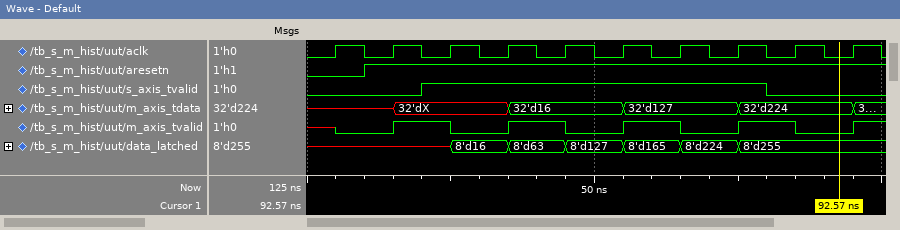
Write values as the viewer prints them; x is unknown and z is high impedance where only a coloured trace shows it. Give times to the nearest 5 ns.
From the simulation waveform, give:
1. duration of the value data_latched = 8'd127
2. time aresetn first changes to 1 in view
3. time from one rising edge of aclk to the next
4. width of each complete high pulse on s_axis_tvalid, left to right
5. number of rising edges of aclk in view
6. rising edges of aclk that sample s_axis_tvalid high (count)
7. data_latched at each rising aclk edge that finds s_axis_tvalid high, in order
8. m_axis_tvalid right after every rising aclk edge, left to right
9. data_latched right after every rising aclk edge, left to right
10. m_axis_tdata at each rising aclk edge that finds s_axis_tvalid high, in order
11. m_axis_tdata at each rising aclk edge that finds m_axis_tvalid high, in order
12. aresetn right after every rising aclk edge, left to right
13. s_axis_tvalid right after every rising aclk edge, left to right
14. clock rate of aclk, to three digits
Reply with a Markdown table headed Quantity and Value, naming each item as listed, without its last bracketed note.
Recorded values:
| Quantity | Value |
|---|---|
| duration of the value data_latched = 8'd127 | 10 ns |
| time aresetn first changes to 1 in view | 10 ns |
| time from one rising edge of aclk to the next | 10 ns |
| width of each complete high pulse on s_axis_tvalid, left to right | 60 ns |
| number of rising edges of aclk in view | 10 |
| rising edges of aclk that sample s_axis_tvalid high | 6 |
| data_latched at each rising aclk edge that finds s_axis_tvalid high, in order | x, 8'd16, 8'd63, 8'd127, 8'd165, 8'd224 |
| m_axis_tvalid right after every rising aclk edge, left to right | 0 1 0 1 0 1 0 1 0 1 |
| data_latched right after every rising aclk edge, left to right | x, x, 8'd16, 8'd63, 8'd127, 8'd165, 8'd224, 8'd255, 8'd255, 8'd255 |
| m_axis_tdata at each rising aclk edge that finds s_axis_tvalid high, in order | 32'dX, 32'dX, 32'd16, 32'd16, 32'd127, 32'd127 |
| m_axis_tdata at each rising aclk edge that finds m_axis_tvalid high, in order | 32'dX, 32'd16, 32'd127, 32'd224 |
| aresetn right after every rising aclk edge, left to right | 0 1 1 1 1 1 1 1 1 1 |
| s_axis_tvalid right after every rising aclk edge, left to right | 0 0 1 1 1 1 1 1 0 0 |
| clock rate of aclk, to three digits | 100 MHz |
